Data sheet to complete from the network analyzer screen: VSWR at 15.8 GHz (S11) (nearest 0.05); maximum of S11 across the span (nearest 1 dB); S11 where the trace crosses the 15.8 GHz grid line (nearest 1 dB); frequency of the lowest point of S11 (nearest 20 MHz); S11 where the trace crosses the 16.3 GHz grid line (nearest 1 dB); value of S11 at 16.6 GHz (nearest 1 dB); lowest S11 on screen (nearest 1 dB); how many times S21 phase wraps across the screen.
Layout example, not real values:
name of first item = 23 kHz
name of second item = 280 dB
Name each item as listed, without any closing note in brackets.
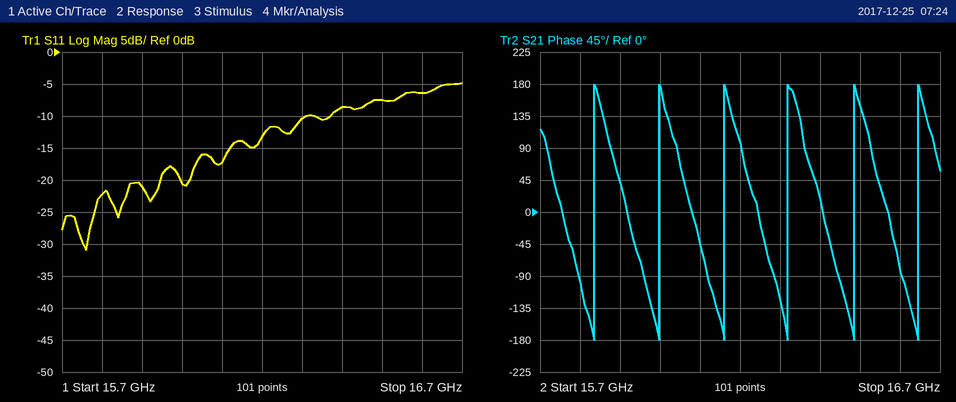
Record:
VSWR at 15.8 GHz (S11) = 1.15
maximum of S11 across the span = -5 dB
S11 where the trace crosses the 15.8 GHz grid line = -22 dB
frequency of the lowest point of S11 = 15.76 GHz
S11 where the trace crosses the 16.3 GHz grid line = -10 dB
value of S11 at 16.6 GHz = -6 dB
lowest S11 on screen = -31 dB
how many times S21 phase wraps across the screen = 6
